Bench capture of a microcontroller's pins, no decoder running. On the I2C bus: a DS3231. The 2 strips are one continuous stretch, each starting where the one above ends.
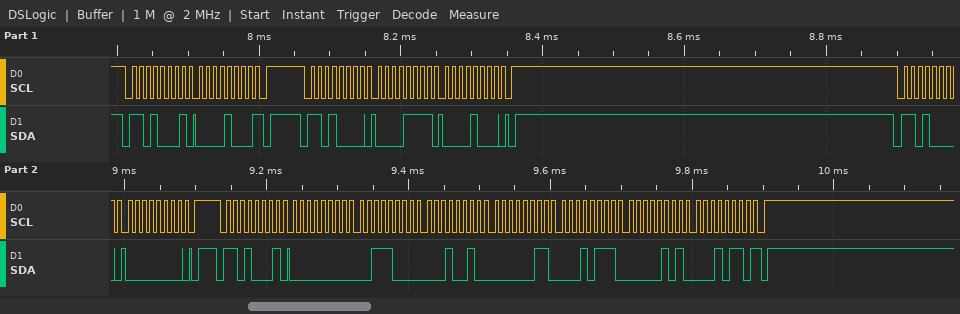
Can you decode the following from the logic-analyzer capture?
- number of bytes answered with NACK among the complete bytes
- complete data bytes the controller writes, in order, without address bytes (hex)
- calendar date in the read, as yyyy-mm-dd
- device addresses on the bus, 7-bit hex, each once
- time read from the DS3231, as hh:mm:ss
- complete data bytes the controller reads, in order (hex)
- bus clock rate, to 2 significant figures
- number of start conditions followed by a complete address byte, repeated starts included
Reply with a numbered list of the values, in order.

1. 2
2. 0F 08 00
3. 2016-05-17
4. 0x68
5. 12:38:00
6. 08 00 38 12 03 17 05 16
7. 100 kHz
8. 4
